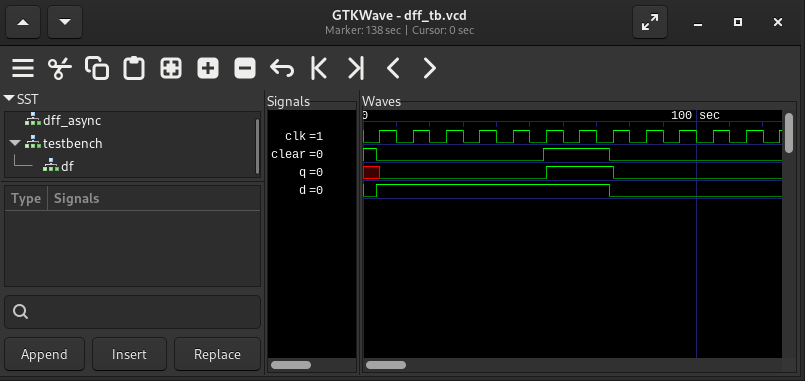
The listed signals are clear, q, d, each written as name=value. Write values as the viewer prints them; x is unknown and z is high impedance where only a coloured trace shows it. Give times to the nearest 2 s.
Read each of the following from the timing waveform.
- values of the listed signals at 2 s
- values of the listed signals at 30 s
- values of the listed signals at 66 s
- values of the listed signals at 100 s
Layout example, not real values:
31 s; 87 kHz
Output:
clear=1, q=x, d=0; clear=0, q=0, d=1; clear=1, q=1, d=1; clear=0, q=0, d=0
